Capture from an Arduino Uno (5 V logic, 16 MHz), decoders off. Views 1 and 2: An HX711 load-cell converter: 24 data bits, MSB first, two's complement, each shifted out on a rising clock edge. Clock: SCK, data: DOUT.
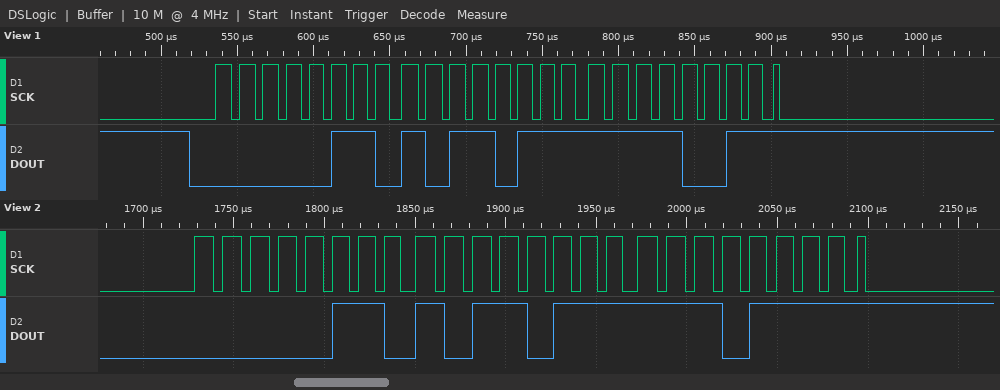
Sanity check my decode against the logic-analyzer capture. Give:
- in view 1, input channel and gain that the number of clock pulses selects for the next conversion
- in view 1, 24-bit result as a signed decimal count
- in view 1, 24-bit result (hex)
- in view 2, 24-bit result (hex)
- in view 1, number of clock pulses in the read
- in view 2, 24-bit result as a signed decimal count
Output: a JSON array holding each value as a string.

["channel A, gain 128", "440307", "0x06B7F3", "0x06B7EF", "25", "440303"]
